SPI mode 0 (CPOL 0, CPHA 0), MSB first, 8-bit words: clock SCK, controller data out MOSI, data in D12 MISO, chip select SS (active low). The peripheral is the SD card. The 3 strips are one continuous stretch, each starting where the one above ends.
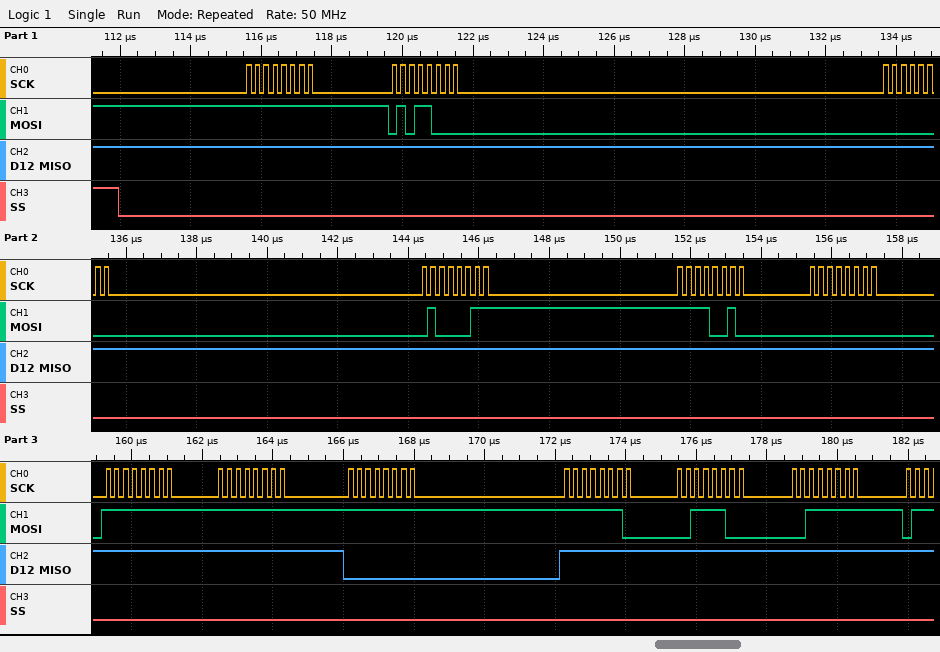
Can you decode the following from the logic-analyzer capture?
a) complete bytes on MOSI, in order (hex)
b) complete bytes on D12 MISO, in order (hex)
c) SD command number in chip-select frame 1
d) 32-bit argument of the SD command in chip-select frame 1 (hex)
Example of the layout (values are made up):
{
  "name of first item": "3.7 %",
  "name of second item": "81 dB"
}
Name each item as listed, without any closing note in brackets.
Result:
{
  "complete bytes on MOSI, in order": "FF 58 00 43 F2 00 FF FF FF FE 3C 3F",
  "complete bytes on D12 MISO, in order": "FF FF FF FF FF FF FF FF 00 FF FF FF",
  "SD command number in chip-select frame 1": "CMD24",
  "32-bit argument of the SD command in chip-select frame 1": "0x0043F200"
}
